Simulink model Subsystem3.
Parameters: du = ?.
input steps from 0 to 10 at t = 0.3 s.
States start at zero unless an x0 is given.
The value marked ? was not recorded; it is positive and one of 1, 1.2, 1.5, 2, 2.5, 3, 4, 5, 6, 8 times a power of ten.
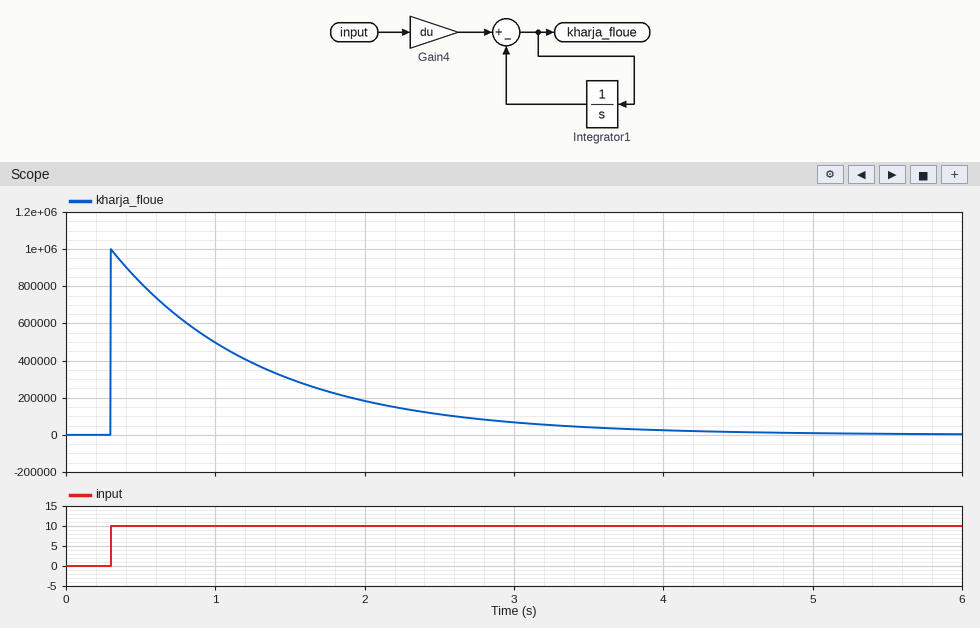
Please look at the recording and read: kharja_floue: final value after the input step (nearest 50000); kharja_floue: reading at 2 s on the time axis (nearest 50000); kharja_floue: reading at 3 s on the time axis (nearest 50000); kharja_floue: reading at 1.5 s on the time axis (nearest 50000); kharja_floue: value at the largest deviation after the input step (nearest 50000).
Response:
0
200000
50000
300000
1000000
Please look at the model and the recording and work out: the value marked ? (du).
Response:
100000
